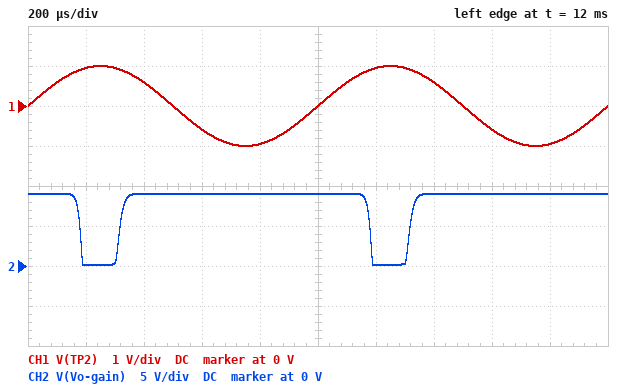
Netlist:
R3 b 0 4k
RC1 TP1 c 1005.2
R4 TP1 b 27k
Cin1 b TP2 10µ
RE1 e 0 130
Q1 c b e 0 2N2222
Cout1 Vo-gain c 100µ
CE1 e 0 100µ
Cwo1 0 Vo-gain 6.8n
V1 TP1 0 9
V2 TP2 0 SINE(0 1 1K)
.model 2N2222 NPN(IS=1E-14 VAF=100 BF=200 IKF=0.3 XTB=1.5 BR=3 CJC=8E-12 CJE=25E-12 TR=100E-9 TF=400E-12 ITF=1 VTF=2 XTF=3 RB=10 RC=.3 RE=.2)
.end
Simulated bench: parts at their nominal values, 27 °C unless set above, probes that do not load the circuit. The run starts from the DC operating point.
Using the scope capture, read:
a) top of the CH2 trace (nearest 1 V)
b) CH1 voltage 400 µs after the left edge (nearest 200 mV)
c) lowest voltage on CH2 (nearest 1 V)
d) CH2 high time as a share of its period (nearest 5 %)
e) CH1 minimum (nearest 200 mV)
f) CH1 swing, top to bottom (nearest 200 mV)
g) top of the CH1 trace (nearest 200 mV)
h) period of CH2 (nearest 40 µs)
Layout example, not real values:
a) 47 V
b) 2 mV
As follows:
a) 9 V
b) 600 mV
c) 0 V
d) 85 %
e) -1.0 V
f) 2.0 V
g) 1.0 V
h) 1.00 ms
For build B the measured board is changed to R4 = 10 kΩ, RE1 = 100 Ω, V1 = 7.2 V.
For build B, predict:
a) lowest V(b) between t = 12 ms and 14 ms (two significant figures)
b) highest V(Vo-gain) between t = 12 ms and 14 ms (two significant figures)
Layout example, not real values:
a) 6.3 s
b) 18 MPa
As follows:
a) -1.0 V
b) 7.2 V
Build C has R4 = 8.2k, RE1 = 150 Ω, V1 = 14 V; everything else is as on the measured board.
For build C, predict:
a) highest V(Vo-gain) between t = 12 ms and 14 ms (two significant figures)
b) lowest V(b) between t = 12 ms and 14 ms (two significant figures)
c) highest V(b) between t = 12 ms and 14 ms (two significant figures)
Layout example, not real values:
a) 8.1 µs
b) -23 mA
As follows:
a) 14 V
b) -730 mV
c) 1.3 V
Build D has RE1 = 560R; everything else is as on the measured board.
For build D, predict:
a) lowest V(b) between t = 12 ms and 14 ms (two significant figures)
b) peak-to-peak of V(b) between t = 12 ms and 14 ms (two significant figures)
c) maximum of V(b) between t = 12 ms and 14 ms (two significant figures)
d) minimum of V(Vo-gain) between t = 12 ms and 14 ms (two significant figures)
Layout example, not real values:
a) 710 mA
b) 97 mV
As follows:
a) -1.0 V
b) 2.0 V
c) 970 mV
d) 210 mV
